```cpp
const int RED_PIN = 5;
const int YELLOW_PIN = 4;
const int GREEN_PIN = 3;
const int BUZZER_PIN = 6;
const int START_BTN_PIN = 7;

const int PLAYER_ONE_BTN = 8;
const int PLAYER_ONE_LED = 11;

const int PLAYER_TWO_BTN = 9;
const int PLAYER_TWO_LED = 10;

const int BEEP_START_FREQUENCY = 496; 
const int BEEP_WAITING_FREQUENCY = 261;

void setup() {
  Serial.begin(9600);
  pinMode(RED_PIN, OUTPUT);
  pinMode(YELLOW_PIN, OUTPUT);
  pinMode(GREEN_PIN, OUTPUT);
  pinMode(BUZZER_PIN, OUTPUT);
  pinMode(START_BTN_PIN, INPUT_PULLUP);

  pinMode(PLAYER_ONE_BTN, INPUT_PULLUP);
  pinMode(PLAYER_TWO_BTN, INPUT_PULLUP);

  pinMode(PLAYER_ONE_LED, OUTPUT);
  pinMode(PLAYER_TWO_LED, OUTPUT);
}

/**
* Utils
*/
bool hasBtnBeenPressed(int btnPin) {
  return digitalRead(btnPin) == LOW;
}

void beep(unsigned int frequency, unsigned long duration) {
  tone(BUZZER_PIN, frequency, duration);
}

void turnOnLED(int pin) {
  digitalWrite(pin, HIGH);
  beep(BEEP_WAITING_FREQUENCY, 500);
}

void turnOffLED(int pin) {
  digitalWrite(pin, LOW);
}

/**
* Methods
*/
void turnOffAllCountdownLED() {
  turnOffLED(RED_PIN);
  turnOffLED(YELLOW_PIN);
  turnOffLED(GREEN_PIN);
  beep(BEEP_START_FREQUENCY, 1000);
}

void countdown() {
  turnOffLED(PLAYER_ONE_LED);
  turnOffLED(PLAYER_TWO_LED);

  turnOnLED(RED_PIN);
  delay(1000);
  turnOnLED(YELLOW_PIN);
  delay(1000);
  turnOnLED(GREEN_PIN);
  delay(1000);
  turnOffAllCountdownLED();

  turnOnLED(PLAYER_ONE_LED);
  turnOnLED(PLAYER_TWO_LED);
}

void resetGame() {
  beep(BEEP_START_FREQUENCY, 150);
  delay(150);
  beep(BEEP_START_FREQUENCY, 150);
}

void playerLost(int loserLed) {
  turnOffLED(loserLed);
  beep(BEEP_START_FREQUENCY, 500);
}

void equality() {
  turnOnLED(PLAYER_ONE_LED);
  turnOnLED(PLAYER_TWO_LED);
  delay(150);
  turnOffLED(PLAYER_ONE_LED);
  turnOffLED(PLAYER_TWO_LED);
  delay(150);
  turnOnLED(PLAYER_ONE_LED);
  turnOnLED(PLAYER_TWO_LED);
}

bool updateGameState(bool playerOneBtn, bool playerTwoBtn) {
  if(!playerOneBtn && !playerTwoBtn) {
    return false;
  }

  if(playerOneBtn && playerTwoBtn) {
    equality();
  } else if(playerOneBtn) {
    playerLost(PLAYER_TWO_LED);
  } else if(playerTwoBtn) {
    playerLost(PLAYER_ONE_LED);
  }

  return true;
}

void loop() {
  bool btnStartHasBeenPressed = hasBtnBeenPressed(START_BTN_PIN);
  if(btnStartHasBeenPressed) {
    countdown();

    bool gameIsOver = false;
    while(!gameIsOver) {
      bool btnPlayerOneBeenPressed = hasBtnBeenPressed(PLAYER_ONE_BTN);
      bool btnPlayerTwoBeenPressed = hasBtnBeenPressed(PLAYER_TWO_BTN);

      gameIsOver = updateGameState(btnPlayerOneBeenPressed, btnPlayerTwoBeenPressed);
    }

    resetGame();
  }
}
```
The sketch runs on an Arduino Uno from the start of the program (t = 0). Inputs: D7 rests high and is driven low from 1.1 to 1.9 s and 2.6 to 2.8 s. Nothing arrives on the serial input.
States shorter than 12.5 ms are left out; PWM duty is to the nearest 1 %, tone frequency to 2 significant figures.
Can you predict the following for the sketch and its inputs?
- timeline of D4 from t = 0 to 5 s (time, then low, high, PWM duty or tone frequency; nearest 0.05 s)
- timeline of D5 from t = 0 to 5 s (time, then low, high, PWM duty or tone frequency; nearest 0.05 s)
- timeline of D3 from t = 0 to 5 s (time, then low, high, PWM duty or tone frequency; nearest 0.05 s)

0 s low; 2.1 s high; 4.1 s low
0 s low; 1.1 s high; 4.1 s low
0 s low; 3.1 s high; 4.1 s low
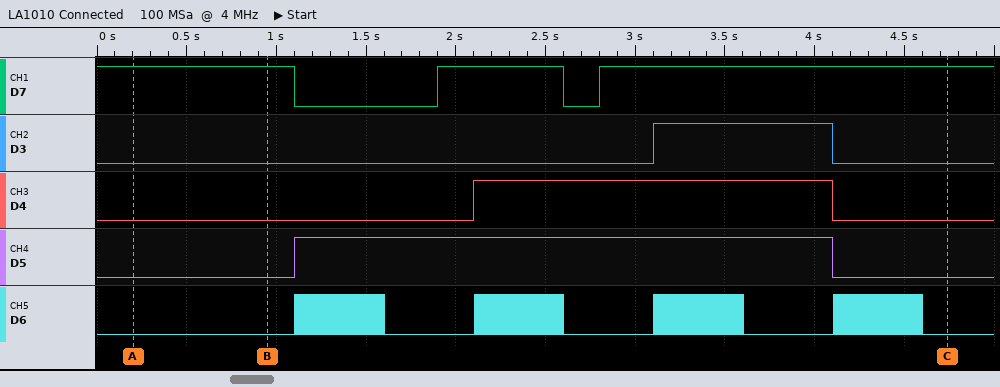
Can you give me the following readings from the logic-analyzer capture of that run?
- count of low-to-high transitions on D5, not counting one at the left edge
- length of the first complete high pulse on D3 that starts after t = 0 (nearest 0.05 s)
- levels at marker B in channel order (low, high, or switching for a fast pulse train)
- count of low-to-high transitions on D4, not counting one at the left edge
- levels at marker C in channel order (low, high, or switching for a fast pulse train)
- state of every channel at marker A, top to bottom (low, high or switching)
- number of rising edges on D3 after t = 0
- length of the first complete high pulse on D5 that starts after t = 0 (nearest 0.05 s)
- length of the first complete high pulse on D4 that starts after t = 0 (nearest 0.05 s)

1
1.00 s
D7 high, D3 low, D4 low, D5 low, D6 low
1
D7 high, D3 low, D4 low, D5 low, D6 low
D7 high, D3 low, D4 low, D5 low, D6 low
1
3.00 s
2.00 s
